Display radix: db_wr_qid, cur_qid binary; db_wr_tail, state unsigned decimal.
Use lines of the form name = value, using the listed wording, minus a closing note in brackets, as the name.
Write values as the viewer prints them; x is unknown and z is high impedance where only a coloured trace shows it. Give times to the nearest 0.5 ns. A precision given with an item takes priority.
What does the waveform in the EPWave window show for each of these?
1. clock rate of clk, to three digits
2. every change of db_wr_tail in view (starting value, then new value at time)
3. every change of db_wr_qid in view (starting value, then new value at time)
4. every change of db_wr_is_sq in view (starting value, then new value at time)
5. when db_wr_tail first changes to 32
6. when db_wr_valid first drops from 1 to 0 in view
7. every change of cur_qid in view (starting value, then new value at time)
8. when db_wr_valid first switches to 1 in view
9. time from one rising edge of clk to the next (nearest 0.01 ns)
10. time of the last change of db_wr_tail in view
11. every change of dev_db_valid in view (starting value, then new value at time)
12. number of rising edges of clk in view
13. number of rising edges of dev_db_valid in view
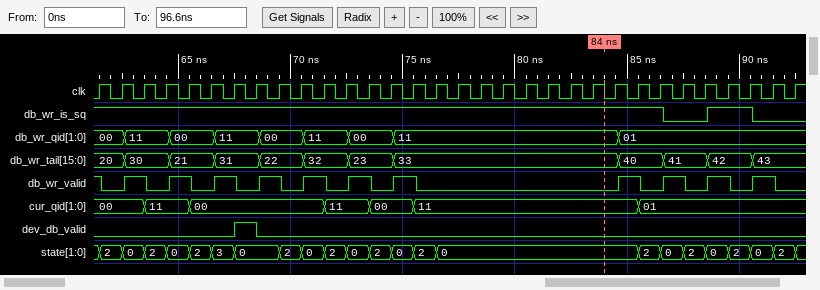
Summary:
clock rate of clk, to three digits = 1.00 GHz
every change of db_wr_tail in view = 20, 30 at 62.5 ns, 21 at 64.5 ns, 31 at 66.5 ns, 22 at 68.5 ns, 32 at 70.5 ns, 23 at 72.5 ns, 33 at 74.5 ns, 40 at 84.5 ns, 41 at 86.5 ns, 42 at 88.5 ns, 43 at 90.5 ns
every change of db_wr_qid in view = 00, 11 at 62.5 ns, 00 at 64.5 ns, 11 at 66.5 ns, 00 at 68.5 ns, 11 at 70.5 ns, 00 at 72.5 ns, 11 at 74.5 ns, 01 at 84.5 ns
every change of db_wr_is_sq in view = 1, 0 at 86.5 ns, 1 at 88.5 ns, 0 at 90.5 ns
when db_wr_tail first changes to 32 = 70.5 ns
when db_wr_valid first drops from 1 to 0 in view = 61.5 ns
every change of cur_qid in view = 00, 11 at 63.5 ns, 00 at 65.5 ns, 11 at 71.5 ns, 00 at 73.5 ns, 11 at 75.5 ns, 01 at 85.5 ns
when db_wr_valid first switches to 1 in view = 62.5 ns
time from one rising edge of clk to the next = 1 ns
time of the last change of db_wr_tail in view = 90.5 ns
every change of dev_db_valid in view = 0, 1 at 67.5 ns, 0 at 68.5 ns
number of rising edges of clk in view = 32
number of rising edges of dev_db_valid in view = 1
